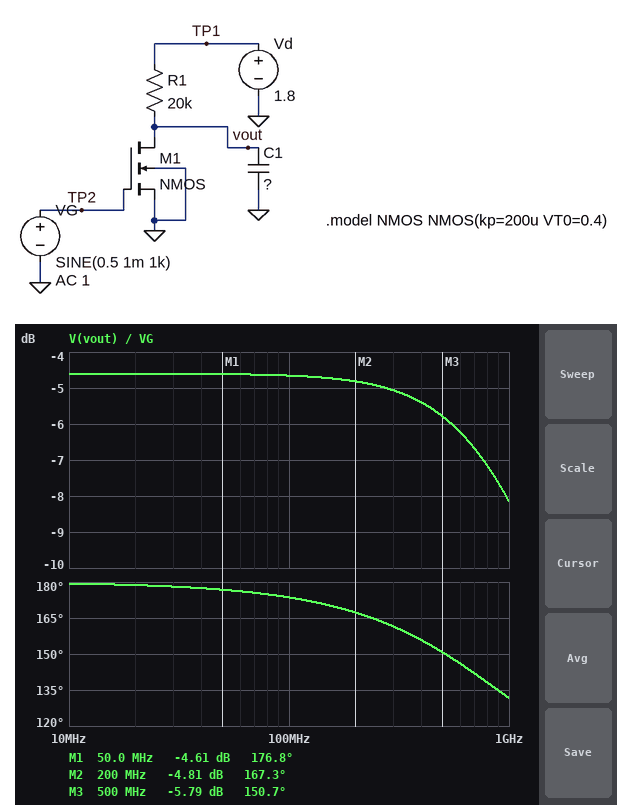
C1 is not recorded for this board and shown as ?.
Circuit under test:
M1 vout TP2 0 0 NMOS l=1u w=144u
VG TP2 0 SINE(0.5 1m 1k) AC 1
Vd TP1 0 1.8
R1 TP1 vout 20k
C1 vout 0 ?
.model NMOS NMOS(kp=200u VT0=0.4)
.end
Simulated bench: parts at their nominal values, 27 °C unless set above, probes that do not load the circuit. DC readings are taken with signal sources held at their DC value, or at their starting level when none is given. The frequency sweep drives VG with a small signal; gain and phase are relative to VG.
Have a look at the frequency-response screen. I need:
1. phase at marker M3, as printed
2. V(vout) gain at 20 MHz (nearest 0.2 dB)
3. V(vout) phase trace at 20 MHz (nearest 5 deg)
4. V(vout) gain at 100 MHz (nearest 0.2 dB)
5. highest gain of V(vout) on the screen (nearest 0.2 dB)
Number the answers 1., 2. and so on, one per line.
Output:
1. 150.7 deg
2. -4.6 dB
3. 180 deg
4. -4.6 dB
5. -4.6 dB
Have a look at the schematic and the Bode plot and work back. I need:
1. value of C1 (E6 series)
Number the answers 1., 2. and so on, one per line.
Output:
1. 330 fF
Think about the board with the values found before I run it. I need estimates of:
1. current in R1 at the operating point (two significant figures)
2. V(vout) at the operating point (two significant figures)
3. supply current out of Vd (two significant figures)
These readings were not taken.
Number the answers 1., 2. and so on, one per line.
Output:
1. 88 µA
2. 38 mV
3. 88 µA
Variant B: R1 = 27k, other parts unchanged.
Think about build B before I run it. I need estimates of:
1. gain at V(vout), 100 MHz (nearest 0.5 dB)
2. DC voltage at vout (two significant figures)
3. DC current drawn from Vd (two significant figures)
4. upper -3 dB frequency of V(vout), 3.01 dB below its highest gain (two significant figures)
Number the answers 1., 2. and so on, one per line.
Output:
1. -9.0 dB
2. 26 mV
3. 66 µA
4. 1.0 GHz
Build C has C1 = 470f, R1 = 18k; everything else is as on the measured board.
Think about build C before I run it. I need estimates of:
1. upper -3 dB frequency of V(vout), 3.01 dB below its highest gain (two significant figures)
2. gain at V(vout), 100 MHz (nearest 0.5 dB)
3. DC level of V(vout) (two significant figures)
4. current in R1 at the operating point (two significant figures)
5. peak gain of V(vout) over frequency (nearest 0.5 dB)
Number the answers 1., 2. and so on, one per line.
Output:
1. 570 MHz
2. -3.0 dB
3. 43 mV
4. 98 µA
5. -2.5 dB
